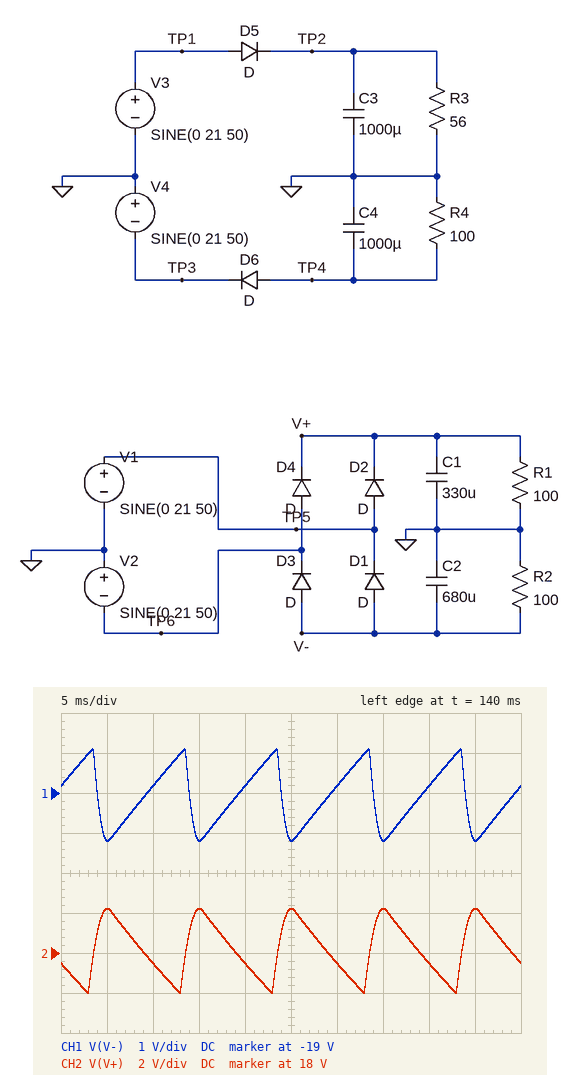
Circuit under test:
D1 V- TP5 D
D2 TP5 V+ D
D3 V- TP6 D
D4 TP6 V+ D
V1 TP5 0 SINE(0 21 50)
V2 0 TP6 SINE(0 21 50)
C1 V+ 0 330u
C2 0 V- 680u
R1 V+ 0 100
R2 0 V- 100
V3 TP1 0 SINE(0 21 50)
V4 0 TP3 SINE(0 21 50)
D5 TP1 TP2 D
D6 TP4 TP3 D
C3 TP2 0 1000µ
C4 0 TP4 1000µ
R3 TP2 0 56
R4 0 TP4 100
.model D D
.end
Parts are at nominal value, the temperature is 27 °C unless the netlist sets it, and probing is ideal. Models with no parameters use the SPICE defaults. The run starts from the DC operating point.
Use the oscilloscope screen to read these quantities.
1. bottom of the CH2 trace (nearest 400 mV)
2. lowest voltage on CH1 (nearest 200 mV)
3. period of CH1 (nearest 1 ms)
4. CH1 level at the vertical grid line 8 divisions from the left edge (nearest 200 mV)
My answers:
16.0 V
-20.2 V
10 ms
-18.8 V
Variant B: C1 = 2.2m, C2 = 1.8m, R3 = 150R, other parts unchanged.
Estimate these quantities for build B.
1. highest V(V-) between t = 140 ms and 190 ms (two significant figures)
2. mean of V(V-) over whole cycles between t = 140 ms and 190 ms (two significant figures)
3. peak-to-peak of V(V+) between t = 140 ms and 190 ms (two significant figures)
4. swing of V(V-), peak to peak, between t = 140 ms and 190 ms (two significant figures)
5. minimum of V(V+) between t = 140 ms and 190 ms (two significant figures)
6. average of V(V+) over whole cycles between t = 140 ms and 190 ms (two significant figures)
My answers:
-19 V
-20 V
800 mV
960 mV
19 V
20 V
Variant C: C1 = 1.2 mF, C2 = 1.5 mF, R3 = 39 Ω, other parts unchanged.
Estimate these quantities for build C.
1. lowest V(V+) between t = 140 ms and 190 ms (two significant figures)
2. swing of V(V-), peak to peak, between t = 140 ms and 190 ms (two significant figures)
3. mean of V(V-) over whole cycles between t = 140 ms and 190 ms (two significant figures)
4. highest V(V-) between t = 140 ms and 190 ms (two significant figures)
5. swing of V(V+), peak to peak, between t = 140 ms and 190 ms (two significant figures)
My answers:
19 V
1.1 V
-20 V
-19 V
1.4 V
